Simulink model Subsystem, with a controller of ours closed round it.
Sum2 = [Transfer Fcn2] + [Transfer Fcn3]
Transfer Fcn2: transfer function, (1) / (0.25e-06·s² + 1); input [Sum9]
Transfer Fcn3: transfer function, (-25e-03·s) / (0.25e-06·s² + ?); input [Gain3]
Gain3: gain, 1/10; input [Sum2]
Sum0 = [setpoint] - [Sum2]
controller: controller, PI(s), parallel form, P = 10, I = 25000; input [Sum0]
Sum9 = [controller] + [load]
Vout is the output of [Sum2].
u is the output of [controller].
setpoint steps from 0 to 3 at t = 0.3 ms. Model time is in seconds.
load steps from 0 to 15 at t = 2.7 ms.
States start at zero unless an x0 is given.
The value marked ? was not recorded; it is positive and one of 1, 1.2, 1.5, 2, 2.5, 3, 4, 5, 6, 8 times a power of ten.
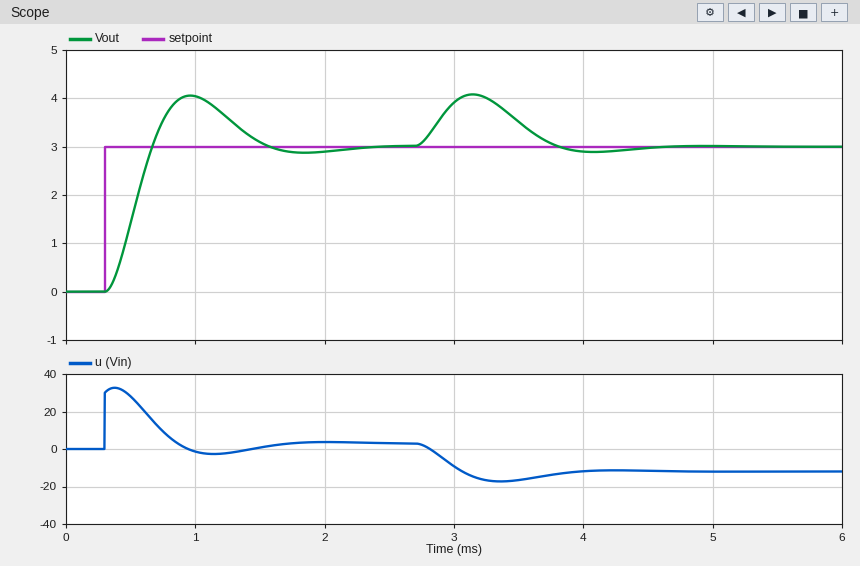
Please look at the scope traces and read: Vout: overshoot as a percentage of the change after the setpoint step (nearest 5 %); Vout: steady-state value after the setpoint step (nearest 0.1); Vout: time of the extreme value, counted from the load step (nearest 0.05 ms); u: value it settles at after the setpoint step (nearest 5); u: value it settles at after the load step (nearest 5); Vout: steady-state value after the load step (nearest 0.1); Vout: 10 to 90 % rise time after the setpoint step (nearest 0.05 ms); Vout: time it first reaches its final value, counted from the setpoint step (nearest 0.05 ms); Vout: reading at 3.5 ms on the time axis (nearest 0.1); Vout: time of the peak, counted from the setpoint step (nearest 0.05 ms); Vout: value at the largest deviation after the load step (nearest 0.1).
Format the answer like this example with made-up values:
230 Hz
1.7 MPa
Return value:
35 %
3.0
0.45 ms
5
-10
3.0
0.25 ms
0.35 ms
3.5
0.65 ms
4.1
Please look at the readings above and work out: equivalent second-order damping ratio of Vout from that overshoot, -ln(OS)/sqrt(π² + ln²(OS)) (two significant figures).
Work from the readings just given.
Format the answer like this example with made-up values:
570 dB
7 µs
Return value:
0.32
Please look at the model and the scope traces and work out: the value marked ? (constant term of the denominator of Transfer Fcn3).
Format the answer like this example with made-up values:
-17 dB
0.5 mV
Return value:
1
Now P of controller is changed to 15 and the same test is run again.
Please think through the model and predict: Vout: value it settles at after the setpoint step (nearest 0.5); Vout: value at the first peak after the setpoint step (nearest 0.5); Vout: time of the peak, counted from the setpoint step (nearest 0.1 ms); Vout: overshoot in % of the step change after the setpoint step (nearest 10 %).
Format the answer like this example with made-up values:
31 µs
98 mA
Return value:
3.0
4.0
0.5 ms
30 %
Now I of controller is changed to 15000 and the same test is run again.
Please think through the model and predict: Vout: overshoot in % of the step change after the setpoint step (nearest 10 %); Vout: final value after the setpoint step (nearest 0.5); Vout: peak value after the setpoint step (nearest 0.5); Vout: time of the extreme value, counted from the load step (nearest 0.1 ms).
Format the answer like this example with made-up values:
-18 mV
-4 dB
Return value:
20 %
3.0
3.5
0.5 ms
